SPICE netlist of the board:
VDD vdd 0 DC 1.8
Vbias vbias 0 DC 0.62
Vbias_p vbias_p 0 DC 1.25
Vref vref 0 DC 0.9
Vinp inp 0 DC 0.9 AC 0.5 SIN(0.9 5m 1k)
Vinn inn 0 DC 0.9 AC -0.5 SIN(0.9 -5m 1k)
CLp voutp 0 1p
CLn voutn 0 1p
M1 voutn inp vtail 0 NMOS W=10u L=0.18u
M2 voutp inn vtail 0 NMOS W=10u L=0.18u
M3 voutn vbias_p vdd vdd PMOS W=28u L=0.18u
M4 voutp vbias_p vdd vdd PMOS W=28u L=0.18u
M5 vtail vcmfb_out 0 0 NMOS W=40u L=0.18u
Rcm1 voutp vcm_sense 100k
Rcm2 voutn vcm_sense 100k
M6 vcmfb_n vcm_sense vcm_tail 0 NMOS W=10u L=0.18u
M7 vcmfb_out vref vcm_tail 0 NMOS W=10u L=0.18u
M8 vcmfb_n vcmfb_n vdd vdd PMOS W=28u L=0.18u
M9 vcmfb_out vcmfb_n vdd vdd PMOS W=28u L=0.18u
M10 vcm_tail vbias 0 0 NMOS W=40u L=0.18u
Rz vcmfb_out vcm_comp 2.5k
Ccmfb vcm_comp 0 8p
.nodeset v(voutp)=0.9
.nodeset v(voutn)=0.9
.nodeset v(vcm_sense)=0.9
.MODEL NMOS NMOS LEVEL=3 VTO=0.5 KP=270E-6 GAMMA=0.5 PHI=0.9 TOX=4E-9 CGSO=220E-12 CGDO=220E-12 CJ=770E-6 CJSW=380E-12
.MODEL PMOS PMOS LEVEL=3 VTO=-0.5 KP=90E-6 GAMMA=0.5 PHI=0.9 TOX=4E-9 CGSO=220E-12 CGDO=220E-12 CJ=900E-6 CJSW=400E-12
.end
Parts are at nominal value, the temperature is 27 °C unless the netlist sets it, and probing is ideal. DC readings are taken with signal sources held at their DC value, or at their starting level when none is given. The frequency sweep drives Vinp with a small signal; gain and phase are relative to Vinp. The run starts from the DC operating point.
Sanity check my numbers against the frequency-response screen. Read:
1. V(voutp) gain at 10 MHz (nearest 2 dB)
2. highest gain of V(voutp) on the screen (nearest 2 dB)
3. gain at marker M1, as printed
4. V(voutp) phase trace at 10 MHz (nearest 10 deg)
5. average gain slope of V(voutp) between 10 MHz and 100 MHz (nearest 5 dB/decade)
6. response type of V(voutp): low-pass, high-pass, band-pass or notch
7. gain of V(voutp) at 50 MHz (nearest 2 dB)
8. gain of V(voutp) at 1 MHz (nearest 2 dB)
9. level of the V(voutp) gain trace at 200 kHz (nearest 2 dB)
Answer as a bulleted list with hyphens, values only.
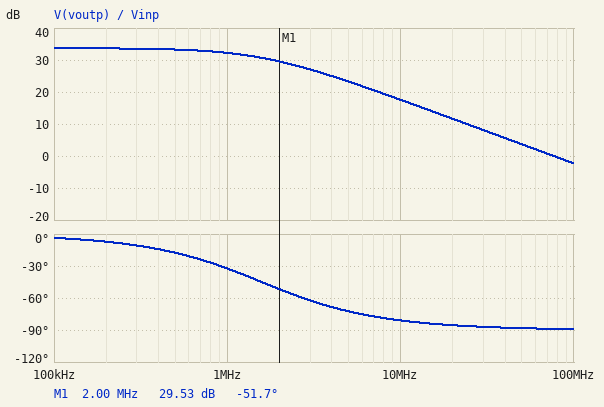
- 18 dB
- 34 dB
- 29.53 dB
- -80 deg
- -20 dB/decade
- low-pass
- 4 dB
- 32 dB
- 34 dB
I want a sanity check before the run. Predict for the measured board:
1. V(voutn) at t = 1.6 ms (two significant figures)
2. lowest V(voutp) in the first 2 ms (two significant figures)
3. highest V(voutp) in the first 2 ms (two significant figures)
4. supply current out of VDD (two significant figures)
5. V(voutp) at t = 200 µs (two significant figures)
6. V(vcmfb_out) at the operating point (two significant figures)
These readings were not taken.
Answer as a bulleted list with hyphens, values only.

- 1.1 V
- 580 mV
- 1.2 V
- 410 µA
- 1.2 V
- 530 mV
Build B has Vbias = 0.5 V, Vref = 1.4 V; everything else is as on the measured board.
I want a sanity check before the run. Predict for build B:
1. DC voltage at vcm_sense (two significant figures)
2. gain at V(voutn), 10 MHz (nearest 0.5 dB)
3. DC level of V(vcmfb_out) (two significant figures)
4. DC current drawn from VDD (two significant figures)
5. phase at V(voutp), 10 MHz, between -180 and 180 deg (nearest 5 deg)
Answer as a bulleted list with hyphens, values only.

- 3.0 mV
- -43.5 dB
- 1.8 V
- 31 µA
- 0 deg
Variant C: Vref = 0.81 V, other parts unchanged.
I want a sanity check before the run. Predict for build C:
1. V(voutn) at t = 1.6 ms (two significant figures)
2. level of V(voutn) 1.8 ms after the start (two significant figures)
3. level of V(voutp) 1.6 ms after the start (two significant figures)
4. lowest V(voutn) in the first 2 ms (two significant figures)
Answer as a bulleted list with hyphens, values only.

- 1.0 V
- 1.1 V
- 620 mV
- 490 mV
